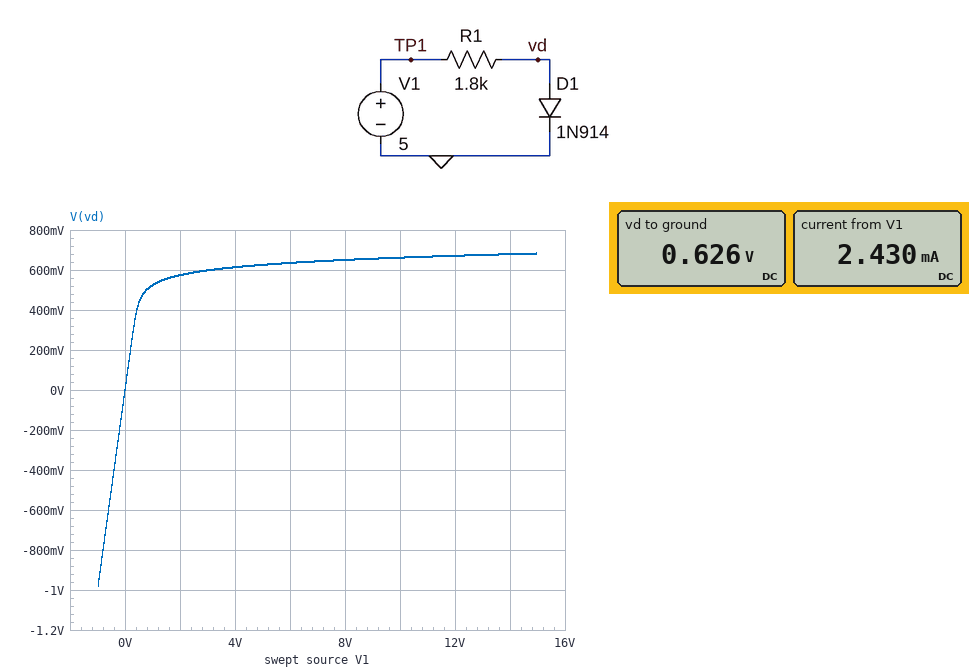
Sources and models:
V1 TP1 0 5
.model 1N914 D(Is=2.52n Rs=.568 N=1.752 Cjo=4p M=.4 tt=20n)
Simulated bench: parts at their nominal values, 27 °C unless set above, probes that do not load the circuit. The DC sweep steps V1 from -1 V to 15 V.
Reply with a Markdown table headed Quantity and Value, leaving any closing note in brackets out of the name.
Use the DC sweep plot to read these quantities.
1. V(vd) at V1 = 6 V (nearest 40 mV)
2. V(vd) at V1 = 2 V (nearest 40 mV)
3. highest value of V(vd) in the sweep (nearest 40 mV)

| Quantity | Value |
|---|---|
| V(vd) at V1 = 6 V | 640 mV |
| V(vd) at V1 = 2 V | 560 mV |
| highest value of V(vd) in the sweep | 680 mV |
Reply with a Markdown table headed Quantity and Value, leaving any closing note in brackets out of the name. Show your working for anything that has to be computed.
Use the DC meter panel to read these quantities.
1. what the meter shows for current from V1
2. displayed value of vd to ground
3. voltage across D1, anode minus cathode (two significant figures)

| Quantity | Value |
|---|---|
| what the meter shows for current from V1 | 2.430 mA |
| displayed value of vd to ground | 0.626 V |
| voltage across D1, anode minus cathode | 626 mV = 630 mV |
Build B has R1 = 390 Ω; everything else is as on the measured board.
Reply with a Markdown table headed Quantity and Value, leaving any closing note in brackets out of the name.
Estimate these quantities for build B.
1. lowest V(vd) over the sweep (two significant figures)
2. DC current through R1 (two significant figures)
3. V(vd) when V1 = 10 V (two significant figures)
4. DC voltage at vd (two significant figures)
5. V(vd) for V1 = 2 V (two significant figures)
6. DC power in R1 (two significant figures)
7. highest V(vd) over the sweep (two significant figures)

| Quantity | Value |
|---|---|
| lowest V(vd) over the sweep | -1.0 V |
| DC current through R1 | 11 mA |
| V(vd) when V1 = 10 V | 740 mV |
| DC voltage at vd | 700 mV |
| V(vd) for V1 = 2 V | 640 mV |
| DC power in R1 | 47 mW |
| highest V(vd) over the sweep | 770 mV |
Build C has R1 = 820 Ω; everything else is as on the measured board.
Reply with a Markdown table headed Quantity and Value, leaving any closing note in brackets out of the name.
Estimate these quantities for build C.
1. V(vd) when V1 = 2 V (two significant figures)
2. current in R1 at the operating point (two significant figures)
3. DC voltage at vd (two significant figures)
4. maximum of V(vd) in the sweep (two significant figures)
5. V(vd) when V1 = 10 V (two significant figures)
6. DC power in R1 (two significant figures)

| Quantity | Value |
|---|---|
| V(vd) when V1 = 2 V | 610 mV |
| current in R1 at the operating point | 5.3 mA |
| DC voltage at vd | 660 mV |
| maximum of V(vd) in the sweep | 720 mV |
| V(vd) when V1 = 10 V | 700 mV |
| DC power in R1 | 23 mW |
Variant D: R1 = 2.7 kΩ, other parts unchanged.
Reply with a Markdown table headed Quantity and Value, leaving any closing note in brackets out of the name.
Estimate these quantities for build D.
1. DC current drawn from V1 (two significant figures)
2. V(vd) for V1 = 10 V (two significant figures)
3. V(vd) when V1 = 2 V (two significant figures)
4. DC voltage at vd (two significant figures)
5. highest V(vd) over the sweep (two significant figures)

| Quantity | Value |
|---|---|
| DC current drawn from V1 | 1.6 mA |
| V(vd) for V1 = 10 V | 640 mV |
| V(vd) when V1 = 2 V | 560 mV |
| DC voltage at vd | 610 mV |
| highest V(vd) over the sweep | 660 mV |
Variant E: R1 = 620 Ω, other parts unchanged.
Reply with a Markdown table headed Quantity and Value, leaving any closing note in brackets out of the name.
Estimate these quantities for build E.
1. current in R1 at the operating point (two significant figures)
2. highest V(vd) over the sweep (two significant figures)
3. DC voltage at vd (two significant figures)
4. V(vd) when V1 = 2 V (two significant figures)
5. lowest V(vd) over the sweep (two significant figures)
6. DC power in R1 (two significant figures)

| Quantity | Value |
|---|---|
| current in R1 at the operating point | 7.0 mA |
| highest V(vd) over the sweep | 740 mV |
| DC voltage at vd | 680 mV |
| V(vd) when V1 = 2 V | 620 mV |
| lowest V(vd) over the sweep | -1.0 V |
| DC power in R1 | 30 mW |
